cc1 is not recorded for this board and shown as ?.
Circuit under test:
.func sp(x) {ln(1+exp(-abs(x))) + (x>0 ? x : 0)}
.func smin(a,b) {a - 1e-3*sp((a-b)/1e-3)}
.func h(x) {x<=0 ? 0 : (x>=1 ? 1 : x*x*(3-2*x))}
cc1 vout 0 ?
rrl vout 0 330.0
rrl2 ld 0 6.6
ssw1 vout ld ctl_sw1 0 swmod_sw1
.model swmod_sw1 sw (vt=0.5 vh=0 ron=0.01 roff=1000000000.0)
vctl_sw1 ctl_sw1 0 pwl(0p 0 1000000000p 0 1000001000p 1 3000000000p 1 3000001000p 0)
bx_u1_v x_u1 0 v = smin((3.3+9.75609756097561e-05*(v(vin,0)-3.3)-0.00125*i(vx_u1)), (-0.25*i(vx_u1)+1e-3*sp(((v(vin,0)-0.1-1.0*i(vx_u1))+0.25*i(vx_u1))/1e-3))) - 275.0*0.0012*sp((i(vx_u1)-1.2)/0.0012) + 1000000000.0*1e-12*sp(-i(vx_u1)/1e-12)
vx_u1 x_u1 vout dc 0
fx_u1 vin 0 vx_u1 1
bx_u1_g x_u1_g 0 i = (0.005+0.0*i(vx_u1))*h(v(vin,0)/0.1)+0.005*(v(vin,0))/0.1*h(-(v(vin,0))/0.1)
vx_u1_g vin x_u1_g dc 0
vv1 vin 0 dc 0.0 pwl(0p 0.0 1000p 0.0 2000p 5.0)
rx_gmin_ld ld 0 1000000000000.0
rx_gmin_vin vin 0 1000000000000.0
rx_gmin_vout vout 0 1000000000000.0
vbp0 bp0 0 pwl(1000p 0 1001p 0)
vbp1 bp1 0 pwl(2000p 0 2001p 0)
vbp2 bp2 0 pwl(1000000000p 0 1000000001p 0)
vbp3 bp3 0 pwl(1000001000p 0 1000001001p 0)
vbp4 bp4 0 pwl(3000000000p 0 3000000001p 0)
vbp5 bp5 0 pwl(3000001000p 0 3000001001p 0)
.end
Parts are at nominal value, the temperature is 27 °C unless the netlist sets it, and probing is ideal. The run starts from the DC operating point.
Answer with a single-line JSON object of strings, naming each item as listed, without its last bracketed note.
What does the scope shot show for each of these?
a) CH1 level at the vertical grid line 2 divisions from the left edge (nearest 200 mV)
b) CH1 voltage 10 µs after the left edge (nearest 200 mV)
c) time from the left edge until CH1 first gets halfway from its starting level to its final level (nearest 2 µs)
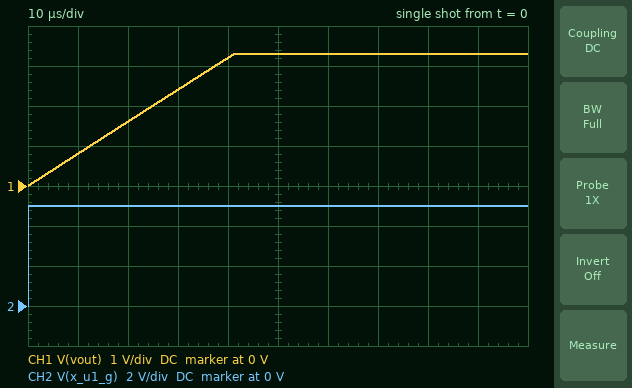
{"CH1 level at the vertical grid line 2 divisions from the left edge": "1.6 V", "CH1 voltage 10 µs after the left edge": "800 mV", "time from the left edge until CH1 first gets halfway from its starting level to its final level": "20 µs"}
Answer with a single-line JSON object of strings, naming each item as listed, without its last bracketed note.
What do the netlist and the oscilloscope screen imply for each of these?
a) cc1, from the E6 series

{"cc1, from the E6 series": "15 µF"}
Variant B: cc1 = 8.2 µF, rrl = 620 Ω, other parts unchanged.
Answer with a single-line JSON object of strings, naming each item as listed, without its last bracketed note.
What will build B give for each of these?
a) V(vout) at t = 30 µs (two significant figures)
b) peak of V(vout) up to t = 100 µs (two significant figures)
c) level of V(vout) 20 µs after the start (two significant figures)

{"V(vout) at t = 30 µs": "3.3 V", "peak of V(vout) up to t = 100 µs": "3.3 V", "level of V(vout) 20 µs after the start": "2.9 V"}
